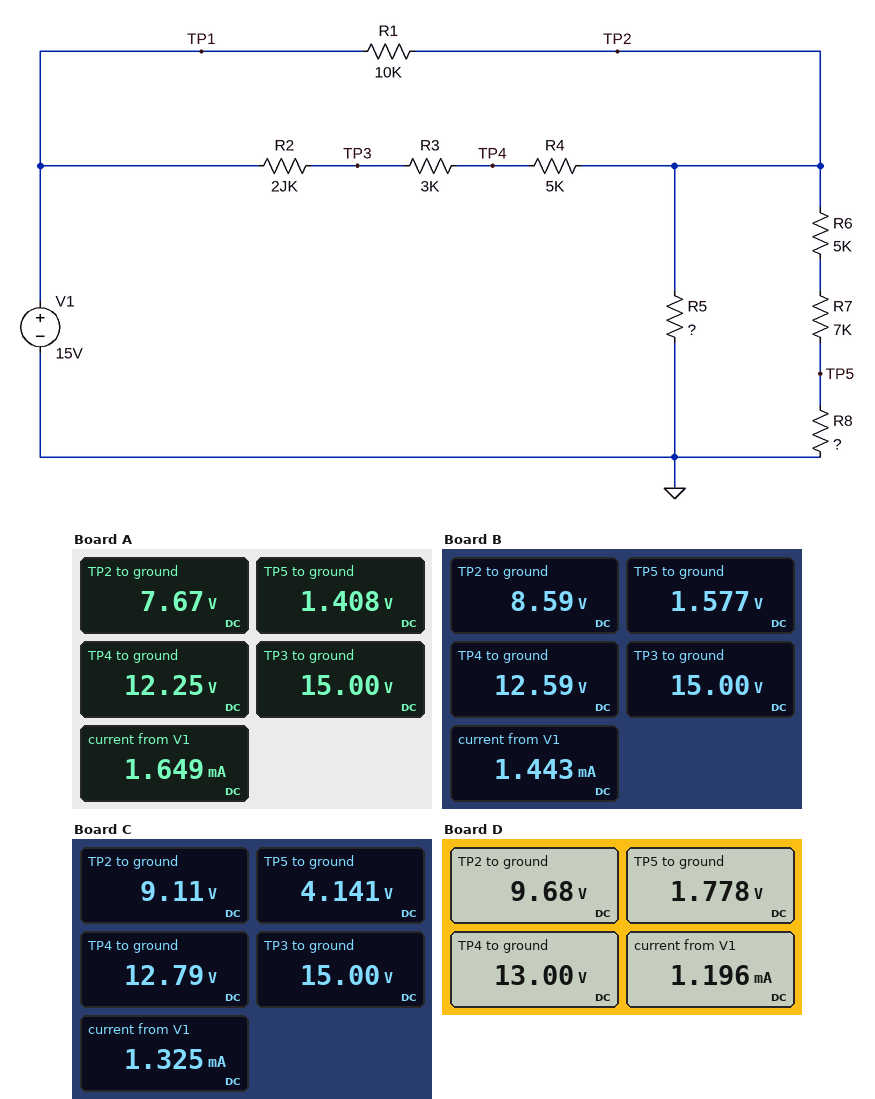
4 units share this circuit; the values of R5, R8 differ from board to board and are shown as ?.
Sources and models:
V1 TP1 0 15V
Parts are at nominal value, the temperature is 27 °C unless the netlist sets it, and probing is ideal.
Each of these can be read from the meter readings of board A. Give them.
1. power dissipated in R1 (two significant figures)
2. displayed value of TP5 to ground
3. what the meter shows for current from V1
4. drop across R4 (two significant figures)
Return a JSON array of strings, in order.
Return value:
["5.4 mW", "1.408 V", "1.649 mA", "4.6 V"]
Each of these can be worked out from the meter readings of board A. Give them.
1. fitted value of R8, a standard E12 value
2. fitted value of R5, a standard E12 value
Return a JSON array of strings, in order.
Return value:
["2.7 kΩ", "6.8 kΩ"]
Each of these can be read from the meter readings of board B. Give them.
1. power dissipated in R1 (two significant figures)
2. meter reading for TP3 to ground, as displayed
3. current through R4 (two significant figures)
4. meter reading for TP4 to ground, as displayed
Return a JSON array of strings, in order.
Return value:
["4.1 mW", "15.00 V", "800 µA", "12.59 V"]
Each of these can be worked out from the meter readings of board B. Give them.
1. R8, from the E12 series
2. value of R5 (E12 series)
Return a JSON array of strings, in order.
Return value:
["2.7 kΩ", "10 kΩ"]
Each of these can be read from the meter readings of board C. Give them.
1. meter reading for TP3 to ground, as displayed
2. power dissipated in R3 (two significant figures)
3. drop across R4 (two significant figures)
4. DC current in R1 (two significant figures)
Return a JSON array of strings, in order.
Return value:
["15.00 V", "1.6 mW", "3.7 V", "590 µA"]
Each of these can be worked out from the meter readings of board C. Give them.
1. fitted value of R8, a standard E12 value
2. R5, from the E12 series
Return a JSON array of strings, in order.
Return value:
["10 kΩ", "10 kΩ"]
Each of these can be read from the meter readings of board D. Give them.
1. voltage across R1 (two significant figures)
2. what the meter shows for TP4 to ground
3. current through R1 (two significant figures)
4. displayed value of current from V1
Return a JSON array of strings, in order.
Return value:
["5.3 V", "13.00 V", "530 µA", "1.196 mA"]
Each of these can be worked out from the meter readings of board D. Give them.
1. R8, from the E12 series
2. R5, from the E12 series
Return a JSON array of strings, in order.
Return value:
["2.7 kΩ", "18 kΩ"]
